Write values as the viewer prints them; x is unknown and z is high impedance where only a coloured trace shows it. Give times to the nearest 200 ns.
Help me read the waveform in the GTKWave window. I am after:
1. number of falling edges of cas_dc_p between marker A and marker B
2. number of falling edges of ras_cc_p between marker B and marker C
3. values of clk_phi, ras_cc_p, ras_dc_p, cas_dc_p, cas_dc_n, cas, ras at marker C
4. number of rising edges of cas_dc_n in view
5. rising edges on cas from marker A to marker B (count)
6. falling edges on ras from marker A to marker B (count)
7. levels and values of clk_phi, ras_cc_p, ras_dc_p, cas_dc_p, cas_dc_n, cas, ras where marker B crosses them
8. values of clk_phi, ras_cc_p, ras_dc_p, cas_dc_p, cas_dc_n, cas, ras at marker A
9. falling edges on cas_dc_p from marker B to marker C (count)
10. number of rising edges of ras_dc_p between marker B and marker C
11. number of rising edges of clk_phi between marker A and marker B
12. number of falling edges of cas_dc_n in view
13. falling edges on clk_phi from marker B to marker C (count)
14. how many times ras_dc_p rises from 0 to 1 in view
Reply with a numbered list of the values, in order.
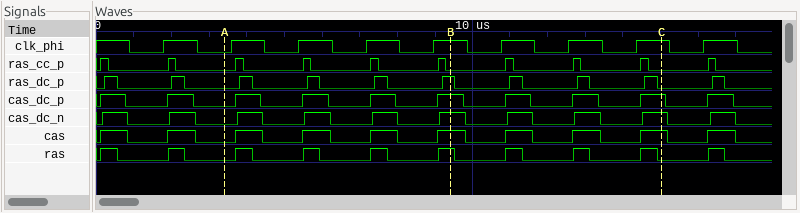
1. 3
2. 3
3. clk_phi=1, ras_cc_p=0, ras_dc_p=0, cas_dc_p=1, cas_dc_n=1, cas=1, ras=0
4. 10
5. 4
6. 3
7. clk_phi=1, ras_cc_p=0, ras_dc_p=1, cas_dc_p=1, cas_dc_n=1, cas=1, ras=1
8. clk_phi=0, ras_cc_p=0, ras_dc_p=0, cas_dc_p=0, cas_dc_n=0, cas=0, ras=0
9. 3
10. 3
11. 4
12. 10
13. 3
14. 10
